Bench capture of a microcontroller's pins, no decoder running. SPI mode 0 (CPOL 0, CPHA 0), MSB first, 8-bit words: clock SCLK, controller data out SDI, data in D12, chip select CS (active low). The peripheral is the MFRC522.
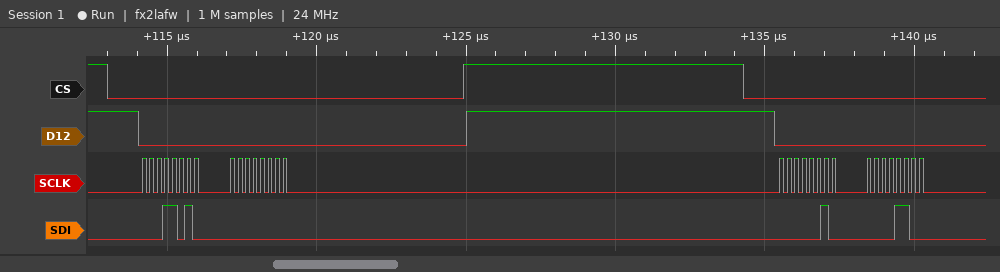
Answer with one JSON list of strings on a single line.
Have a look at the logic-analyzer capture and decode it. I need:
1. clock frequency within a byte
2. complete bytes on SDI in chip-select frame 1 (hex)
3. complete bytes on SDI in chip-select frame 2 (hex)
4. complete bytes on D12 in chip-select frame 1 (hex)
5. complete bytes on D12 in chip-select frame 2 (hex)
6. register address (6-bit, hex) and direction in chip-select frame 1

["4 MHz", "1A 00", "02 0C", "00 00", "00 00", "0x0D write"]
